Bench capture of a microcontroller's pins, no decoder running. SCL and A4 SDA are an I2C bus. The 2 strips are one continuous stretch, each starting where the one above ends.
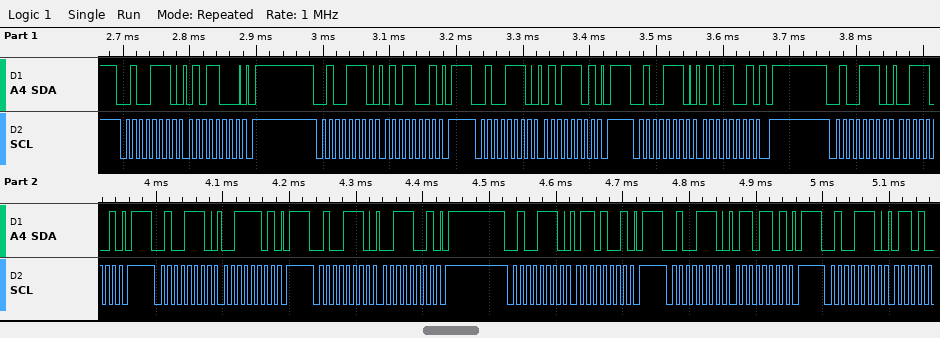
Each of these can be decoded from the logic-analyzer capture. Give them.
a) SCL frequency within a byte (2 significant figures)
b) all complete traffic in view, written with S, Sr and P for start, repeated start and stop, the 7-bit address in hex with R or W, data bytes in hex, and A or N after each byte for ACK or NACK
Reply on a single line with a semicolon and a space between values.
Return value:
100 kHz; S 27W A 58 A P S 27W A 59 A P S 27W A 5D A P S 27W A 59 A P S 27W A 39 A P S 27W A 3D A P S 27W A 39 A P S 27W A 69 A P S 27W A 6D A P S 27W A
